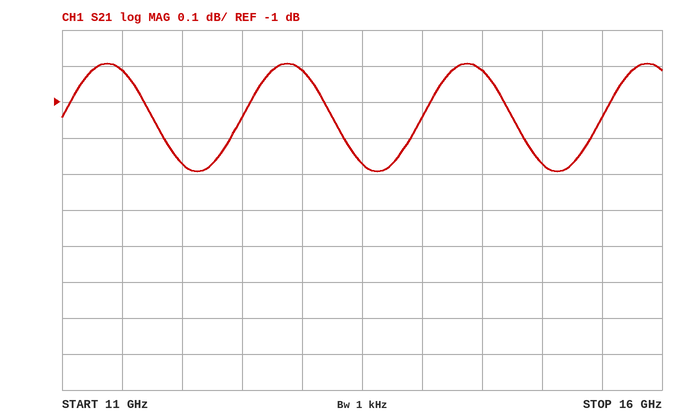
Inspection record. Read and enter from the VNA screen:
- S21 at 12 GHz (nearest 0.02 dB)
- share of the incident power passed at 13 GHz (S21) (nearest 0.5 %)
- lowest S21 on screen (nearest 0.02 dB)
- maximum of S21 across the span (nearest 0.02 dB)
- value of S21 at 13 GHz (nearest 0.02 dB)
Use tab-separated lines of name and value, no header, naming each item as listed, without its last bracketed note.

S21 at 12 GHz	-1.18 dB
share of the incident power passed at 13 GHz (S21)	81.0 %
lowest S21 on screen	-1.20 dB
maximum of S21 across the span	-0.90 dB
value of S21 at 13 GHz	-0.92 dB
